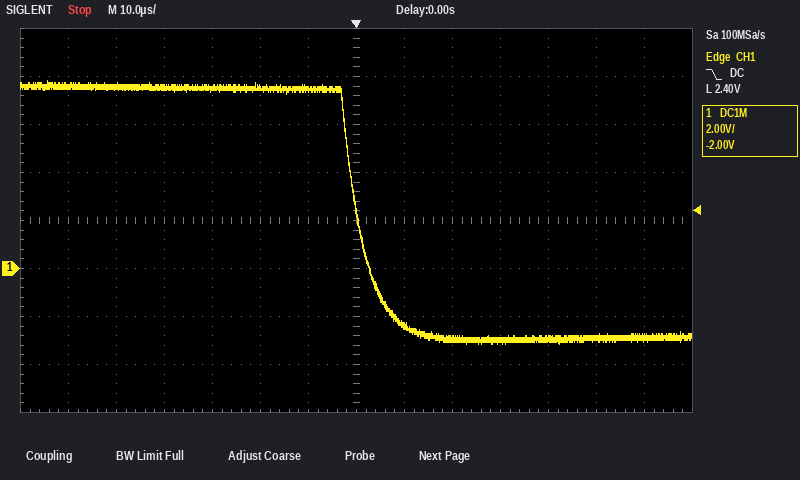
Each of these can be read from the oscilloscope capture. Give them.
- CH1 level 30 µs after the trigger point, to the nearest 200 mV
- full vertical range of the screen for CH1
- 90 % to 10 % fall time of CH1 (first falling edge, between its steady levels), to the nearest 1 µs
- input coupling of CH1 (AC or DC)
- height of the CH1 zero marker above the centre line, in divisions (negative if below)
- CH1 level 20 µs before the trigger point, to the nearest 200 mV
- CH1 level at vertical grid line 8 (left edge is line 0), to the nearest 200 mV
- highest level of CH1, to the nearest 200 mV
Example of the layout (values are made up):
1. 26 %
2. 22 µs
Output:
1. -3.0 V
2. 16 V
3. 10 µs
4. DC
5. -1.0 div
6. 7.6 V
7. -2.4 V
8. 7.8 V
